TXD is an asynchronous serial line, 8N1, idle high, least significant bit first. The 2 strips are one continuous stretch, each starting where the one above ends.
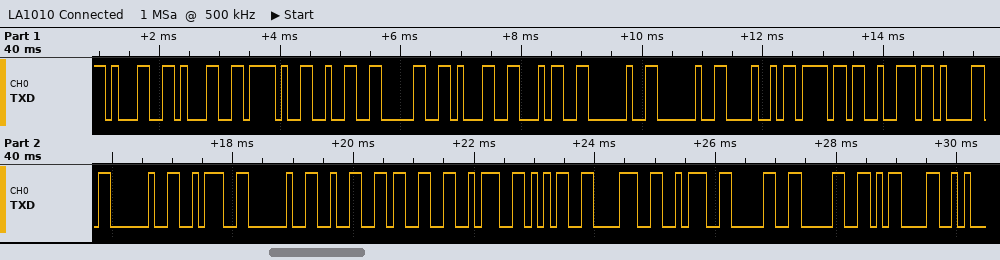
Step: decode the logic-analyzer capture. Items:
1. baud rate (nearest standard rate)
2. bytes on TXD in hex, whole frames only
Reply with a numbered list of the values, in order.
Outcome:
1. 9600 baud
2. 31 31 2F 32 30 31 34 20 20 48 6F 72 61 20 3A 20 32 33 3A 35 38 3A 30 30 0D
